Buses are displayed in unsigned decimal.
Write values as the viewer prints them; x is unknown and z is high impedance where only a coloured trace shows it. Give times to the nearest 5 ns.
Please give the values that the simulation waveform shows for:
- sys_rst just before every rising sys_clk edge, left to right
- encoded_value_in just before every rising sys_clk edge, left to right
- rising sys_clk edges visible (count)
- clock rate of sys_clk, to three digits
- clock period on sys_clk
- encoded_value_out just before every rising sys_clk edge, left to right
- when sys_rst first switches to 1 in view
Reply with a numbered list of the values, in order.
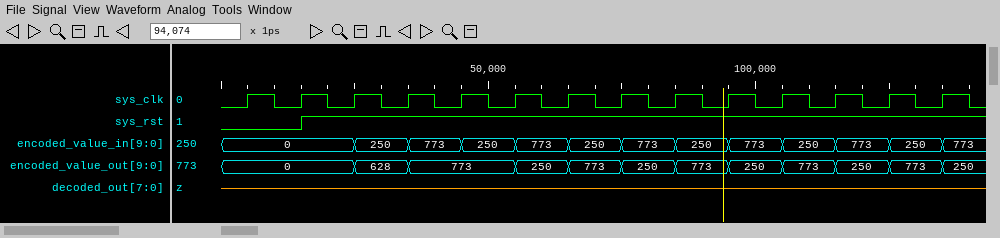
1. 0 0 1 1 1 1 1 1 1 1 1 1 1 1
2. 0, 0, 0, 250, 773, 250, 773, 250, 773, 250, 773, 250, 773, 250
3. 14
4. 100 MHz
5. 10 ns
6. 0, 0, 0, 628, 773, 773, 250, 773, 250, 773, 250, 773, 250, 773
7. 15 ns
